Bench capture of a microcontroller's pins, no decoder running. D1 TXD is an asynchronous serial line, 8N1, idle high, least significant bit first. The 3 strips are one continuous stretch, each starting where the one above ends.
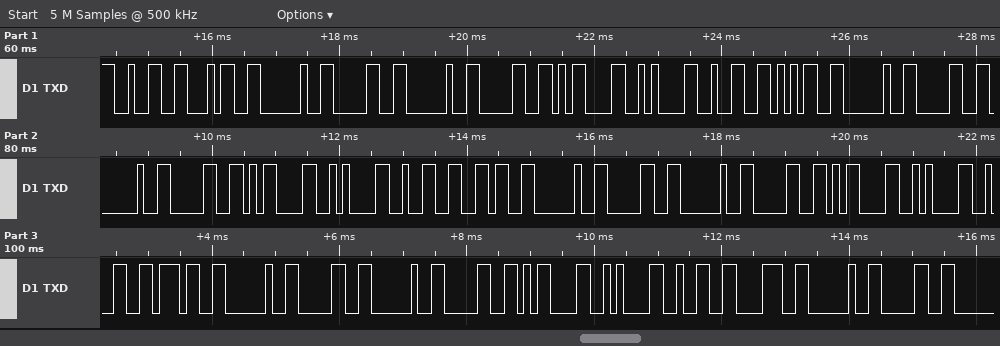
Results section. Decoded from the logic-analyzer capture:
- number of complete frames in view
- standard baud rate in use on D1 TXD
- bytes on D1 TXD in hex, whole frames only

36
9600 baud
32 34 20 30 20 30 0D 0A 32 35 20 30 20 30 0D 0A 32 36 20 30 20 30 0D 0A 32 37 20 30 20 30 0D 0A 32 38 20 30
